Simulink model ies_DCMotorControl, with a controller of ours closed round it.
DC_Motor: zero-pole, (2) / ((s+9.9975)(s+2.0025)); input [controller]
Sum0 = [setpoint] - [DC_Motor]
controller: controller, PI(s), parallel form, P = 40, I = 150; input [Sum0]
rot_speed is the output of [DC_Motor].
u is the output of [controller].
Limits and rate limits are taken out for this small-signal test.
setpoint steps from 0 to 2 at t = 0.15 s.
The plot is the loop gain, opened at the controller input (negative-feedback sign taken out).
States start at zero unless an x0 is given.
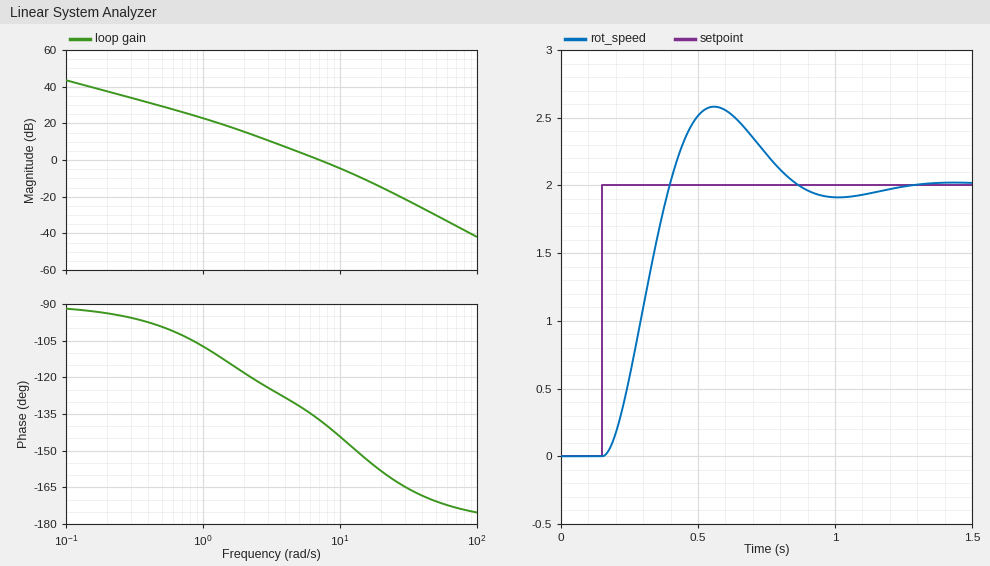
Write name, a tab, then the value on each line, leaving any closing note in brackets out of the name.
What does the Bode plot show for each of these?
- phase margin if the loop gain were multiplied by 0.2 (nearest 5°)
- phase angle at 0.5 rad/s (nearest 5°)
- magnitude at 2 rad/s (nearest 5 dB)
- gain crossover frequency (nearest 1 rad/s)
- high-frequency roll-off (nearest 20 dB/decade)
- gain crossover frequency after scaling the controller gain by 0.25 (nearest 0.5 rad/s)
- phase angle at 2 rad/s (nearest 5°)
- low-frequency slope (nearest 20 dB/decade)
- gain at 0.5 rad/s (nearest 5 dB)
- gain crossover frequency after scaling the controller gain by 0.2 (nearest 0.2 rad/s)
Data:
phase margin if the loop gain were multiplied by 0.2	60°
phase angle at 0.5 rad/s	-100°
magnitude at 2 rad/s	15 dB
gain crossover frequency	7 rad/s
high-frequency roll-off	-40 dB/decade
gain crossover frequency after scaling the controller gain by 0.25	2.5 rad/s
phase angle at 2 rad/s	-120°
low-frequency slope	-20 dB/decade
gain at 0.5 rad/s	30 dB
gain crossover frequency after scaling the controller gain by 0.2	2.2 rad/s
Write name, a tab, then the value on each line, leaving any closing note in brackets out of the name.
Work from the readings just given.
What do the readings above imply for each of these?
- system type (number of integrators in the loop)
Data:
system type	1
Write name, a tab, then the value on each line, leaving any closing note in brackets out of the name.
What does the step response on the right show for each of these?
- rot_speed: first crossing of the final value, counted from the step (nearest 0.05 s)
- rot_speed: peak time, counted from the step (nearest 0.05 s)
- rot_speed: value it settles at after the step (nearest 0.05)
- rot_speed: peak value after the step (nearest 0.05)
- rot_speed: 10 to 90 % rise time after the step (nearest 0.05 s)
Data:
rot_speed: first crossing of the final value, counted from the step	0.25 s
rot_speed: peak time, counted from the step	0.40 s
rot_speed: value it settles at after the step	2.00
rot_speed: peak value after the step	2.60
rot_speed: 10 to 90 % rise time after the step	0.15 s
